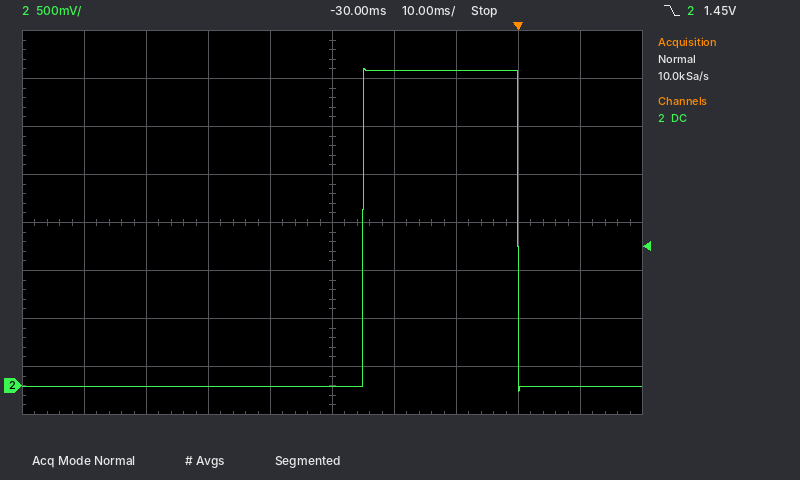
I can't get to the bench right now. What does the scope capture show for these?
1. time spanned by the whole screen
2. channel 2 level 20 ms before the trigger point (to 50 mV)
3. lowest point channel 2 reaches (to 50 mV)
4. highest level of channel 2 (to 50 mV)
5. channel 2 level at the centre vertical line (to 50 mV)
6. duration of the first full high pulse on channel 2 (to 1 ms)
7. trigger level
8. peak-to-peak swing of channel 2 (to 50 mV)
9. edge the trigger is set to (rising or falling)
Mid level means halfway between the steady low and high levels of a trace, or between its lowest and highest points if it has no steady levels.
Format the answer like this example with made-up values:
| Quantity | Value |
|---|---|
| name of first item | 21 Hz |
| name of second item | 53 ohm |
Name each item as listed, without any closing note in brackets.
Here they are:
| Quantity | Value |
|---|---|
| time spanned by the whole screen | 100 ms |
| channel 2 level 20 ms before the trigger point | 3.30 V |
| lowest point channel 2 reaches | -50 mV |
| highest level of channel 2 | 3.30 V |
| channel 2 level at the centre vertical line | 0 mV |
| duration of the first full high pulse on channel 2 | 25 ms |
| trigger level | 1.45 V |
| peak-to-peak swing of channel 2 | 3.35 V |
| edge the trigger is set to | falling |
